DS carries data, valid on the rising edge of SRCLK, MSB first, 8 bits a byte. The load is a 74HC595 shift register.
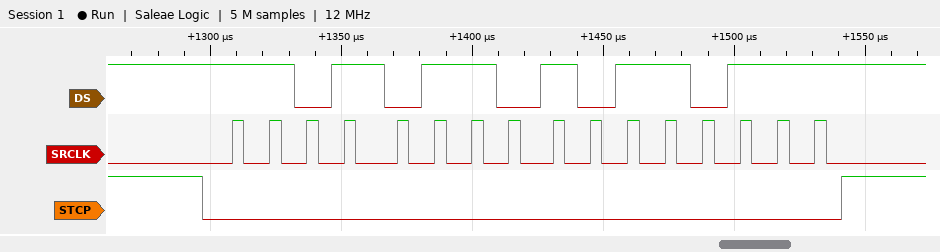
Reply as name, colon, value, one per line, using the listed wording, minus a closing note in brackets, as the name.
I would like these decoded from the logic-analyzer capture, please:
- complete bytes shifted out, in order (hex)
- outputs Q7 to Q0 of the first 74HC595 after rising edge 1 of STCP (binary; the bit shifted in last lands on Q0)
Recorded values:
complete bytes shifted out, in order: D6 B7
outputs Q7 to Q0 of the first 74HC595 after rising edge 1 of STCP: 10110111
